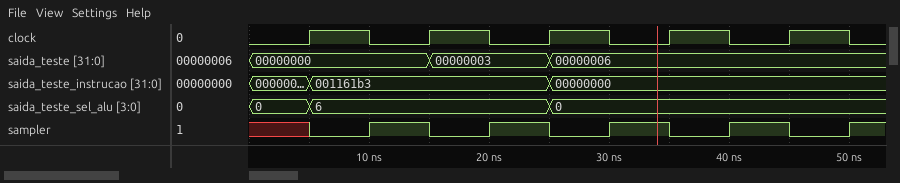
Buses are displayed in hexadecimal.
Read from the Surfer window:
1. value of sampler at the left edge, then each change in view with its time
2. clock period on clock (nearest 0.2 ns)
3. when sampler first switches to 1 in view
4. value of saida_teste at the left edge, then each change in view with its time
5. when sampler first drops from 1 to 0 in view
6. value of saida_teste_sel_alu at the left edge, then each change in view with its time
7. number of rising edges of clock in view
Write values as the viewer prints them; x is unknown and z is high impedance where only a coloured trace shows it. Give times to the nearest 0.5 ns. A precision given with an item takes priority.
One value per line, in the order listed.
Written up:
x, 0 at 5 ns, 1 at 10 ns, 0 at 15 ns, 1 at 20 ns, 0 at 25 ns, 1 at 30 ns, 0 at 35 ns, 1 at 40 ns, 0 at 45 ns, 1 at 50 ns
10 ns
10 ns
00000000, 00000003 at 15 ns, 00000006 at 25 ns
15 ns
0, 6 at 5 ns, 0 at 25 ns
5
